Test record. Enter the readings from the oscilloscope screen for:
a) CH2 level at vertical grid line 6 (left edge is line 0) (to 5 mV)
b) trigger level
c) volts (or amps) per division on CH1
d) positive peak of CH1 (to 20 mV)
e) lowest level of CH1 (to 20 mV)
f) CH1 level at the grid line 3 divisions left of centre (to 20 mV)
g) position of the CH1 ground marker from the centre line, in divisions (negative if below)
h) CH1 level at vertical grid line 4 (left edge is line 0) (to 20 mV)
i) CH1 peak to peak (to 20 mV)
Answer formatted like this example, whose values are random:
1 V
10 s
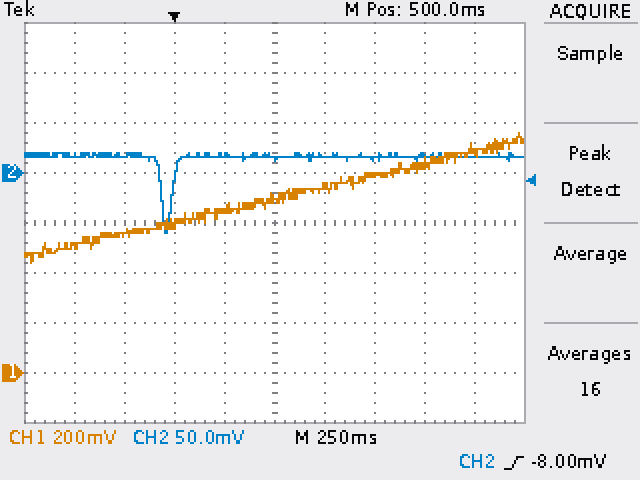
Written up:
15 mV
-8.00 mV
200 mV
960 mV
440 mV
560 mV
-3.0 div
660 mV
520 mV
